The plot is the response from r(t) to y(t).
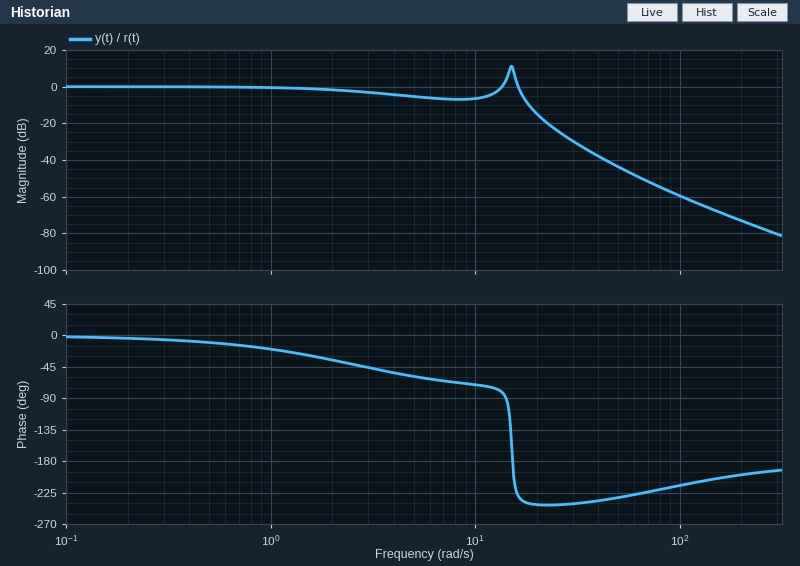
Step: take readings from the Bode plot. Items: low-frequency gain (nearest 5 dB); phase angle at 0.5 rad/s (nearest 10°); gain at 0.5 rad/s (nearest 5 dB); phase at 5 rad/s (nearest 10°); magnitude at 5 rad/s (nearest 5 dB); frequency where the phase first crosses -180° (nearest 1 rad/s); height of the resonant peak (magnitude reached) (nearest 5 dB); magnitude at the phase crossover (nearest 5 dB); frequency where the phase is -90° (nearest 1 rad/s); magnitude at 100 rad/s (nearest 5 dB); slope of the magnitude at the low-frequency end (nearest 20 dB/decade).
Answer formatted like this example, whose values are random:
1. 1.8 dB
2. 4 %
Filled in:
1. 0 dB
2. -10°
3. 0 dB
4. -60°
5. -5 dB
6. 15 rad/s
7. 10 dB
8. 10 dB
9. 14 rad/s
10. -60 dB
11. 0 dB/decade
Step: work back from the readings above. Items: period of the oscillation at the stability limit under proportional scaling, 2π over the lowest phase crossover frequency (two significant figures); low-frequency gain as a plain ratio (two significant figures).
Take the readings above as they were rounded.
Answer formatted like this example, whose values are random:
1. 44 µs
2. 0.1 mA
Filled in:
1. 0.42 s
2. 1.0
